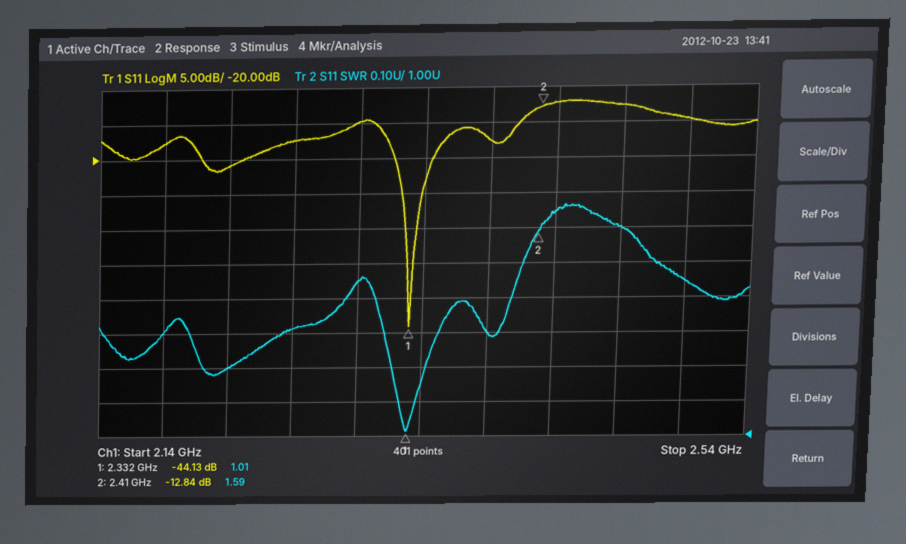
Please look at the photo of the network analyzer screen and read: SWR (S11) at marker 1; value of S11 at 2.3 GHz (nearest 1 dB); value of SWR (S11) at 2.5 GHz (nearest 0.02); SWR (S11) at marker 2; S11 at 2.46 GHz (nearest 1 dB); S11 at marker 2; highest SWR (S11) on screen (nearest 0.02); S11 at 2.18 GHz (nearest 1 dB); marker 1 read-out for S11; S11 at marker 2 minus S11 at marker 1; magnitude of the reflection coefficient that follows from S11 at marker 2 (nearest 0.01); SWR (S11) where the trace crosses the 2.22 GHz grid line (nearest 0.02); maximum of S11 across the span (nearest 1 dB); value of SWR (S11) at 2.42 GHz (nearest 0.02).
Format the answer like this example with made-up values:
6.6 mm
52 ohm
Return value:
1.01
-15 dB
1.44
1.59
-13 dB
-12.84 dB
1.66
-18 dB
-44.13 dB
31.29 dB
0.23
1.20
-12 dB
1.64
